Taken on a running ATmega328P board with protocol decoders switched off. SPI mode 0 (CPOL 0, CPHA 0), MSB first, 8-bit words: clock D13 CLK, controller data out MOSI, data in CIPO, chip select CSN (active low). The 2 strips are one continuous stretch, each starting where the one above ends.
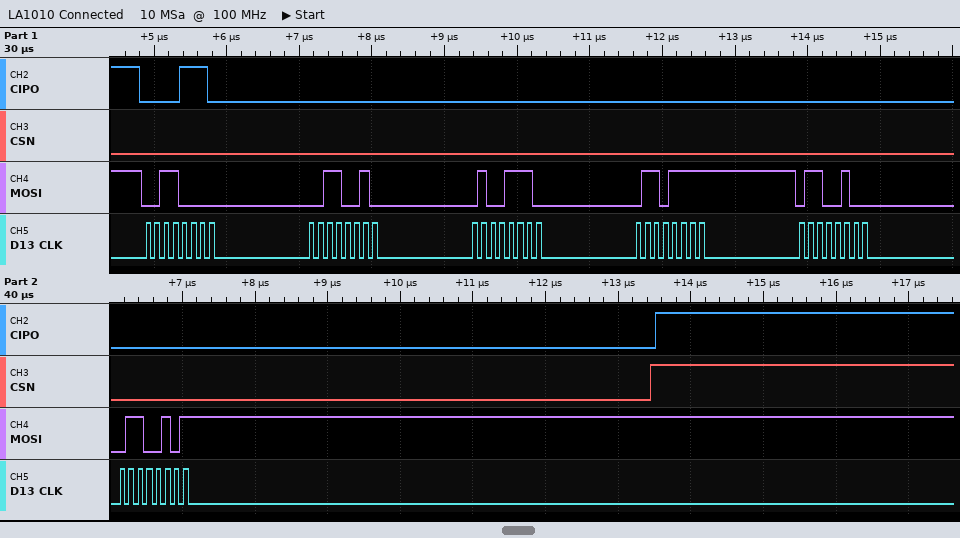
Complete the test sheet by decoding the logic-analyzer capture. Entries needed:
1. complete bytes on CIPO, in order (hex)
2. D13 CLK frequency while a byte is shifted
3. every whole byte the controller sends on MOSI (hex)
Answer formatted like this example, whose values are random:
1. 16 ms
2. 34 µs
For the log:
1. 0E 00 00 00 00 00
2. 8 MHz
3. 30 32 4E 6F 64 65
